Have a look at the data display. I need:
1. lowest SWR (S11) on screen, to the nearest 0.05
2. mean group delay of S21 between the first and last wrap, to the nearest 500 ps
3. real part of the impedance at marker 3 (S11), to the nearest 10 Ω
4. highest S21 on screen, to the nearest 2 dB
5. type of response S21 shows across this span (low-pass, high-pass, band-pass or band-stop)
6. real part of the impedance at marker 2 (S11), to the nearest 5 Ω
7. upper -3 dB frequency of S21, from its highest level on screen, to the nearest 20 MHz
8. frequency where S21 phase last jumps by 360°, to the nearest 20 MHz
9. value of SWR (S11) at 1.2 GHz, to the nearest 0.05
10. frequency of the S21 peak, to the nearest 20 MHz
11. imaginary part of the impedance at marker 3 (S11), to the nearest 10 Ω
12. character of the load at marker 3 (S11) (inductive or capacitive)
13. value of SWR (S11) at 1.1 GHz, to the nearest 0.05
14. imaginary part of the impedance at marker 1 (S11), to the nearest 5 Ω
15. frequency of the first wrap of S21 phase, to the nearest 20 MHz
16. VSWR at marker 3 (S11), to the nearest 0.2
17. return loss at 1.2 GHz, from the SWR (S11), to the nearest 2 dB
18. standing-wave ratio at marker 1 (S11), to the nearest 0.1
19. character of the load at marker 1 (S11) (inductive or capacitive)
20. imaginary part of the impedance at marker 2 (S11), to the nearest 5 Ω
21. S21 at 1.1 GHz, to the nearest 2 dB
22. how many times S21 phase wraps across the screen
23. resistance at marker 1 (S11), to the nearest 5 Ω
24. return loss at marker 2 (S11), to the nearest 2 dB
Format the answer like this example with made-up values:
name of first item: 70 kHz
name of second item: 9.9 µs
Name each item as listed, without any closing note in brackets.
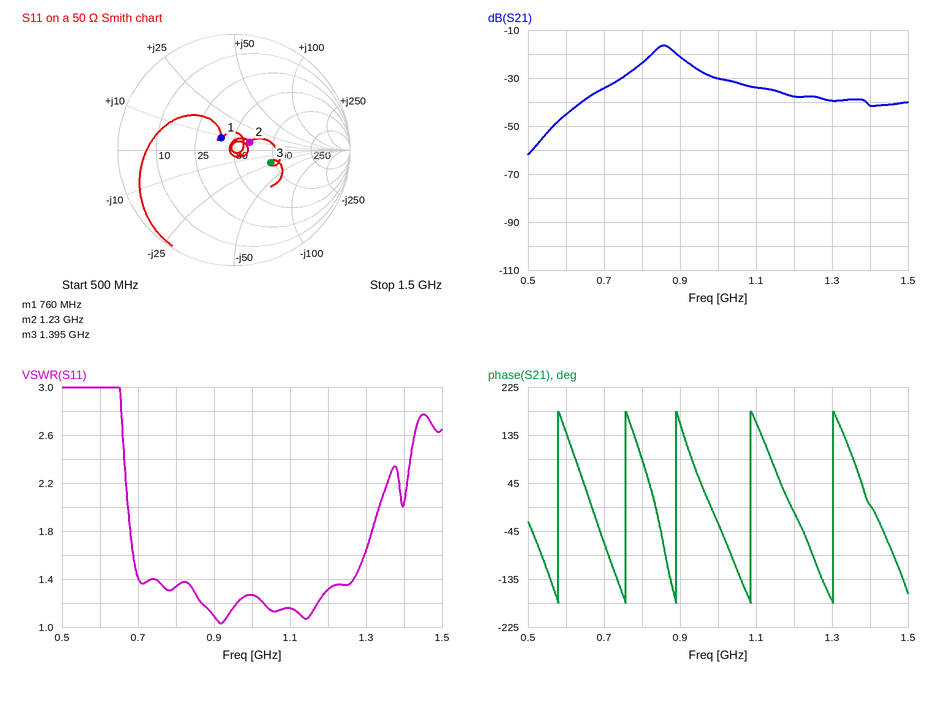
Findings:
lowest SWR (S11) on screen, to the nearest 0.05: 1.05
mean group delay of S21 between the first and last wrap, to the nearest 500 ps: 5.5 ns
real part of the impedance at marker 3 (S11), to the nearest 10 Ω: 90 Ω
highest S21 on screen, to the nearest 2 dB: -16 dB
type of response S21 shows across this span: band-pass
real part of the impedance at marker 2 (S11), to the nearest 5 Ω: 65 Ω
upper -3 dB frequency of S21, from its highest level on screen, to the nearest 20 MHz: 880 MHz
frequency where S21 phase last jumps by 360°, to the nearest 20 MHz: 1.30 GHz
value of SWR (S11) at 1.2 GHz, to the nearest 0.05: 1.30
frequency of the S21 peak, to the nearest 20 MHz: 860 MHz
imaginary part of the impedance at marker 3 (S11), to the nearest 10 Ω: -20 Ω
character of the load at marker 3 (S11): capacitive
value of SWR (S11) at 1.1 GHz, to the nearest 0.05: 1.15
imaginary part of the impedance at marker 1 (S11), to the nearest 5 Ω: +10 Ω
frequency of the first wrap of S21 phase, to the nearest 20 MHz: 580 MHz
VSWR at marker 3 (S11), to the nearest 0.2: 2.0
return loss at 1.2 GHz, from the SWR (S11), to the nearest 2 dB: 18 dB
standing-wave ratio at marker 1 (S11), to the nearest 0.1: 1.4
character of the load at marker 1 (S11): inductive
imaginary part of the impedance at marker 2 (S11), to the nearest 5 Ω: +10 Ω
S21 at 1.1 GHz, to the nearest 2 dB: -34 dB
how many times S21 phase wraps across the screen: 5
resistance at marker 1 (S11), to the nearest 5 Ω: 40 Ω
return loss at marker 2 (S11), to the nearest 2 dB: 16 dB
